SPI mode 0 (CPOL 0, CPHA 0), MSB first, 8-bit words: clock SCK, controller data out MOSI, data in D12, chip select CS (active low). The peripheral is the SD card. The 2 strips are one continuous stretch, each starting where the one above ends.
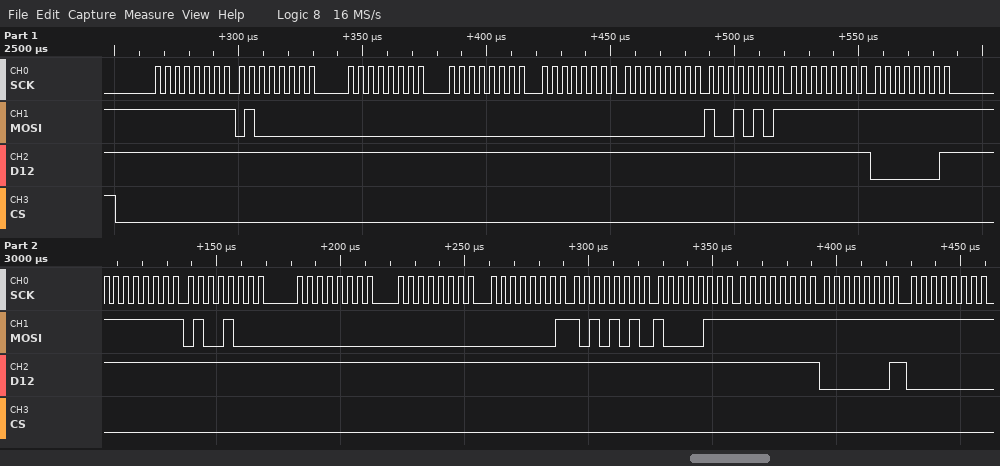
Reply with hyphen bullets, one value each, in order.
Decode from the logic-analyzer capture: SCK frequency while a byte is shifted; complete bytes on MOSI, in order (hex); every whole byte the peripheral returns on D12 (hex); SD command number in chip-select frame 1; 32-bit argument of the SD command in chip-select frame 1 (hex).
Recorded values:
- 250 kHz
- 0xFF 0x40 0x00 0x00 0x00 0x00 0x95 0xFF 0xFF 0xFF 0x48 0x00 0x00 0x01 0xAA 0x87 0xFF 0xFF 0xFF
- 0xFF 0xFF 0xFF 0xFF 0xFF 0xFF 0xFF 0xFF 0x01 0xFF 0xFF 0xFF 0xFF 0xFF 0xFF 0xFF 0xFF 0x01 0x00
- CMD0
- 0x00000000
